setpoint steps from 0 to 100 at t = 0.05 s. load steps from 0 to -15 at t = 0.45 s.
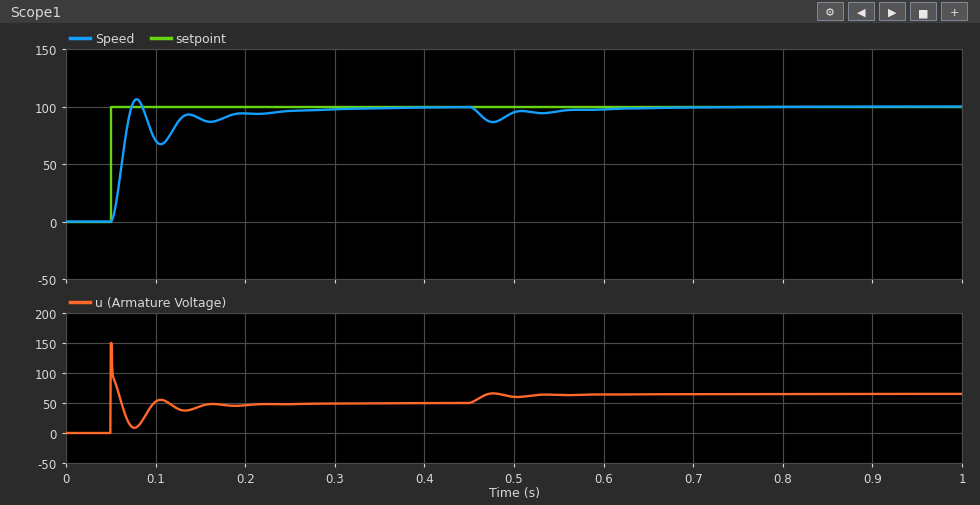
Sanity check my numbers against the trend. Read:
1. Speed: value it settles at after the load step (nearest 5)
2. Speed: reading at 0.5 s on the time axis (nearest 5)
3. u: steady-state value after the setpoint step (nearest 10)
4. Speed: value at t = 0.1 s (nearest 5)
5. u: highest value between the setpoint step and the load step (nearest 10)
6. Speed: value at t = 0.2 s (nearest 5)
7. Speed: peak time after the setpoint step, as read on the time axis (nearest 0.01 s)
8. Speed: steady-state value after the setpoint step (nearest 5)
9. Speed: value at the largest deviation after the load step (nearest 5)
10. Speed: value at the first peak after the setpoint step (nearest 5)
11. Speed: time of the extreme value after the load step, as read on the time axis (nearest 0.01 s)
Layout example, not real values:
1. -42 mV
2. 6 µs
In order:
1. 100
2. 95
3. 50
4. 70
5. 150
6. 95
7. 0.08 s
8. 100
9. 85
10. 105
11. 0.48 s
